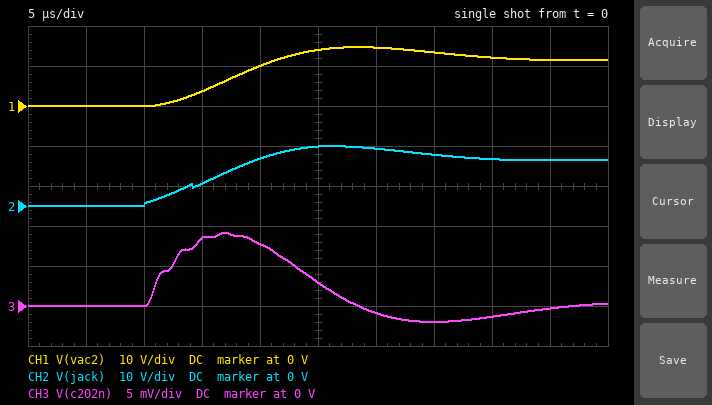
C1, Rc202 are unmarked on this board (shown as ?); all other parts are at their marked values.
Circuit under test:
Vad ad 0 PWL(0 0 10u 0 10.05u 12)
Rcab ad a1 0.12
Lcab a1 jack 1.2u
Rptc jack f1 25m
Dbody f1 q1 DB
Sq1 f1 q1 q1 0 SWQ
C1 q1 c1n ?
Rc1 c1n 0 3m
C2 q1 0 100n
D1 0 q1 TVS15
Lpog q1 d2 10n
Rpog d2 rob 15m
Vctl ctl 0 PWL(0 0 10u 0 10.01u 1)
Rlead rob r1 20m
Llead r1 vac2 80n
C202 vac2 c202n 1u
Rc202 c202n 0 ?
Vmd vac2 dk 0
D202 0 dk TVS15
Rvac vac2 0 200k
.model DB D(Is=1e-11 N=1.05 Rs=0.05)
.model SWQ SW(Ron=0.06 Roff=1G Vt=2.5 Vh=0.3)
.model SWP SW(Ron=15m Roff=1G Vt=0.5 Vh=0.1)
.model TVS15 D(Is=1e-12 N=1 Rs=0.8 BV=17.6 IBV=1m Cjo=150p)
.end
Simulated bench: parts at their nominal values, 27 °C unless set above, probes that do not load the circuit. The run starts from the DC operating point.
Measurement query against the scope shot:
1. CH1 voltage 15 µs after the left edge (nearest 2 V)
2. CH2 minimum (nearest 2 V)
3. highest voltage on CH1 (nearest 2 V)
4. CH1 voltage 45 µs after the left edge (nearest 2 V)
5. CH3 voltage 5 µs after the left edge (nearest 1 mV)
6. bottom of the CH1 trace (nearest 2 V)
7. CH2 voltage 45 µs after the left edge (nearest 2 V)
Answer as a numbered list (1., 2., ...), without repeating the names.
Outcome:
1. 4 V
2. 0 V
3. 14 V
4. 12 V
5. 0 V
6. 0 V
7. 12 V
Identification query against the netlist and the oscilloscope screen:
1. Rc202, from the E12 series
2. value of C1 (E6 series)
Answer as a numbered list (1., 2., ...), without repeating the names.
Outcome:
1. 6.8 mΩ
2. 22 µF
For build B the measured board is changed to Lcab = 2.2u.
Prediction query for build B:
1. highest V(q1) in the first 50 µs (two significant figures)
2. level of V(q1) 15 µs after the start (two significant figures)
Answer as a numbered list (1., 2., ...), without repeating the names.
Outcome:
1. 16 V
2. 2.3 V
